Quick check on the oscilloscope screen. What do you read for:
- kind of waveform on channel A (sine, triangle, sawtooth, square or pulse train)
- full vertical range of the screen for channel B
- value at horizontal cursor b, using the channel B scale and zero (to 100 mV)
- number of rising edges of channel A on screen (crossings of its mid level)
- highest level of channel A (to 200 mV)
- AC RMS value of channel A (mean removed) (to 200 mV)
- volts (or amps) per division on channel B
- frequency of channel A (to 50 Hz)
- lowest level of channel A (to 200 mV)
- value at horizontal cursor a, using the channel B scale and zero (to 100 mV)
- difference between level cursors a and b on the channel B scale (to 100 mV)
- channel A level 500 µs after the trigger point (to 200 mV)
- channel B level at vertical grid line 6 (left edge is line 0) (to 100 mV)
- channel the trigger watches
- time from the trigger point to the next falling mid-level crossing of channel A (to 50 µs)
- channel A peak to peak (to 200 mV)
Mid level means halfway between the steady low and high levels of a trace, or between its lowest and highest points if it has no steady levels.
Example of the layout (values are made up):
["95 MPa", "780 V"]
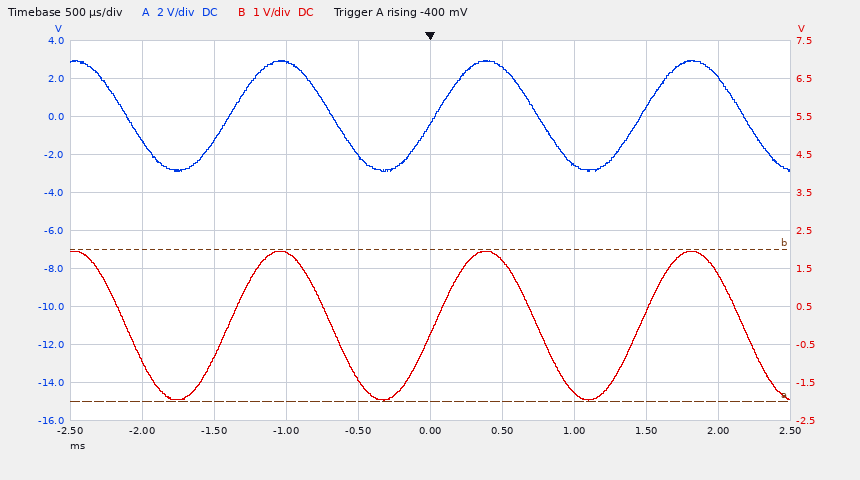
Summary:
["sine", "10 V", "2.0 V", "3", "3.0 V", "2.0 V", "1 V", "700 Hz", "-2.8 V", "-2.0 V", "4.0 V", "2.6 V", "1.7 V", "channel A", "750 µs", "5.8 V"]
